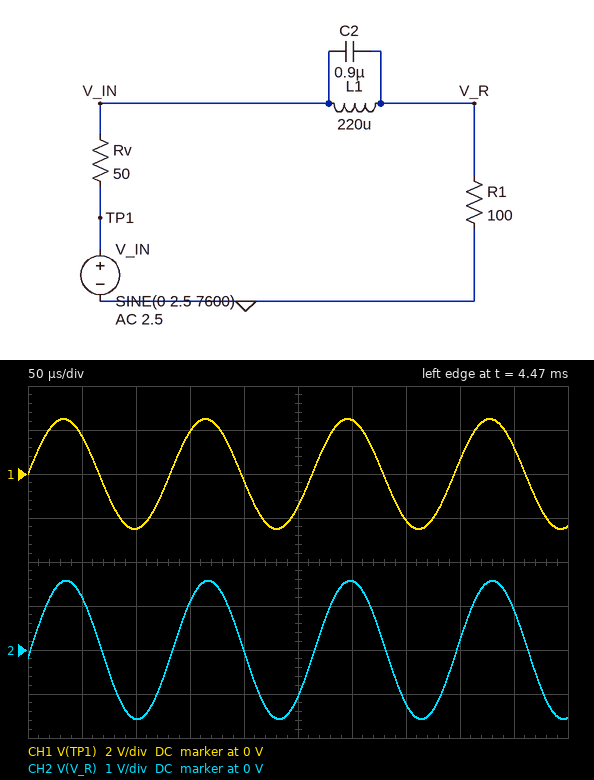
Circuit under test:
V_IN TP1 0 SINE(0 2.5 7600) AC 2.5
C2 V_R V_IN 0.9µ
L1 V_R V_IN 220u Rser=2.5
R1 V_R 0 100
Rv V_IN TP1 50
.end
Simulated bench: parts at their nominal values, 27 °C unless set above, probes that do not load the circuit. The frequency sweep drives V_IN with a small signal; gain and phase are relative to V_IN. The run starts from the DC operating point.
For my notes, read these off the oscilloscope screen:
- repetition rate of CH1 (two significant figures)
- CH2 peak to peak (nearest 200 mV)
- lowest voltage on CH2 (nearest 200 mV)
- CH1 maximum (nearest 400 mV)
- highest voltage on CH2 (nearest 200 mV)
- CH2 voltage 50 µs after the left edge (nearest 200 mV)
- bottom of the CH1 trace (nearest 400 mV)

7.6 kHz
3.2 V
-1.6 V
2.4 V
1.6 V
1.2 V
-2.4 V
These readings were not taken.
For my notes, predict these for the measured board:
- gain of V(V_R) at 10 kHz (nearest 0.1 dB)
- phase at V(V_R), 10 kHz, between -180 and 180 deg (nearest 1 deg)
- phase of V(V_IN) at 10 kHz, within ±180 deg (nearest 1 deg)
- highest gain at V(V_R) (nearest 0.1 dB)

-5.6 dB
-12 deg
4 deg
-3.5 dB
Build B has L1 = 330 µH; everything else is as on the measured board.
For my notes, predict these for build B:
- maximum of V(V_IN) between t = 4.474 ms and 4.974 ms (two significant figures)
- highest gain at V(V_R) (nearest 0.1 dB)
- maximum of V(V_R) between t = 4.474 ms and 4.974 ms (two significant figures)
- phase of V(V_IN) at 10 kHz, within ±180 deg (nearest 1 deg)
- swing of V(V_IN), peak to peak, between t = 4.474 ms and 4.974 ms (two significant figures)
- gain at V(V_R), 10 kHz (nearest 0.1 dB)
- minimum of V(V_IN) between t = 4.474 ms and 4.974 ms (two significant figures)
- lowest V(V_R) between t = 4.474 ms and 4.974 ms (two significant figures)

1.8 V
-3.5 dB
1.4 V
-6 deg
3.6 V
-6.7 dB
-1.8 V
-1.4 V
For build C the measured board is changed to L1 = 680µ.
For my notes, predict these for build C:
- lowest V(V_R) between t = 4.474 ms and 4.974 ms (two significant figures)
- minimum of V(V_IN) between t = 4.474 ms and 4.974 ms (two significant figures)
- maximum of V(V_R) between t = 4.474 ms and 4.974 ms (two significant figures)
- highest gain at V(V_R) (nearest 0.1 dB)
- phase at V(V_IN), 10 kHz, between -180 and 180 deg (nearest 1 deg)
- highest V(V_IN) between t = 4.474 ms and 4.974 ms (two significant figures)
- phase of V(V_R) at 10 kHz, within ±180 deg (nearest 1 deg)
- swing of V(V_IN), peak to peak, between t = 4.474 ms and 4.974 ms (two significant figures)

-1.4 V
-1.9 V
1.4 V
-3.5 dB
-5 deg
1.9 V
11 deg
3.8 V
